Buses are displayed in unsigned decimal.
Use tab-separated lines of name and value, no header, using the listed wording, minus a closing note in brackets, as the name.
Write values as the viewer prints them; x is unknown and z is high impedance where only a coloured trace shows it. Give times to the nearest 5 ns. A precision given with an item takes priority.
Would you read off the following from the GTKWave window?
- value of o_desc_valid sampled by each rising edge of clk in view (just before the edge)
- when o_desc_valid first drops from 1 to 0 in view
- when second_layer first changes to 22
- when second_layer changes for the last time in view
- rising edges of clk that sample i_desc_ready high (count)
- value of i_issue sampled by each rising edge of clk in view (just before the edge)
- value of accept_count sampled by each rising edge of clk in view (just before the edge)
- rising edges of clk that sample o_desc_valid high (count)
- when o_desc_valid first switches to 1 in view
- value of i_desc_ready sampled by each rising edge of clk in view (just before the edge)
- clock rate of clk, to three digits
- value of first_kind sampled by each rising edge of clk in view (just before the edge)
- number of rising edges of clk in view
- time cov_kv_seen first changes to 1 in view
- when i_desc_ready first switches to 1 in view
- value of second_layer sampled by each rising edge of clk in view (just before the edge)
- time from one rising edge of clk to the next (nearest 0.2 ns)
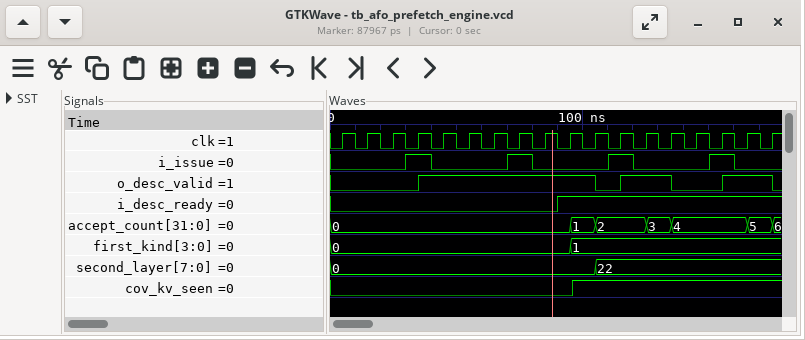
value of o_desc_valid sampled by each rising edge of clk in view	0 0 0 0 1 1 1 1 1 1 1 0 1 1 0 0 1 1
when o_desc_valid first drops from 1 to 0 in view	105 ns
when second_layer first changes to 22	105 ns
when second_layer changes for the last time in view	105 ns
rising edges of clk that sample i_desc_ready high	9
value of i_issue sampled by each rising edge of clk in view	0 0 0 1 0 0 0 1 0 0 0 1 0 0 0 1 0 0
value of accept_count sampled by each rising edge of clk in view	0, 0, 0, 0, 0, 0, 0, 0, 0, 0, 1, 2, 2, 3, 4, 4, 4, 5
rising edges of clk that sample o_desc_valid high	11
when o_desc_valid first switches to 1 in view	35 ns
value of i_desc_ready sampled by each rising edge of clk in view	0 0 0 0 0 0 0 0 0 1 1 1 1 1 1 1 1 1
clock rate of clk, to three digits	100 MHz
value of first_kind sampled by each rising edge of clk in view	0, 0, 0, 0, 0, 0, 0, 0, 0, 0, 1, 1, 1, 1, 1, 1, 1, 1
number of rising edges of clk in view	18
time cov_kv_seen first changes to 1 in view	95 ns
when i_desc_ready first switches to 1 in view	90 ns
value of second_layer sampled by each rising edge of clk in view	0, 0, 0, 0, 0, 0, 0, 0, 0, 0, 0, 22, 22, 22, 22, 22, 22, 22
time from one rising edge of clk to the next	10 ns
